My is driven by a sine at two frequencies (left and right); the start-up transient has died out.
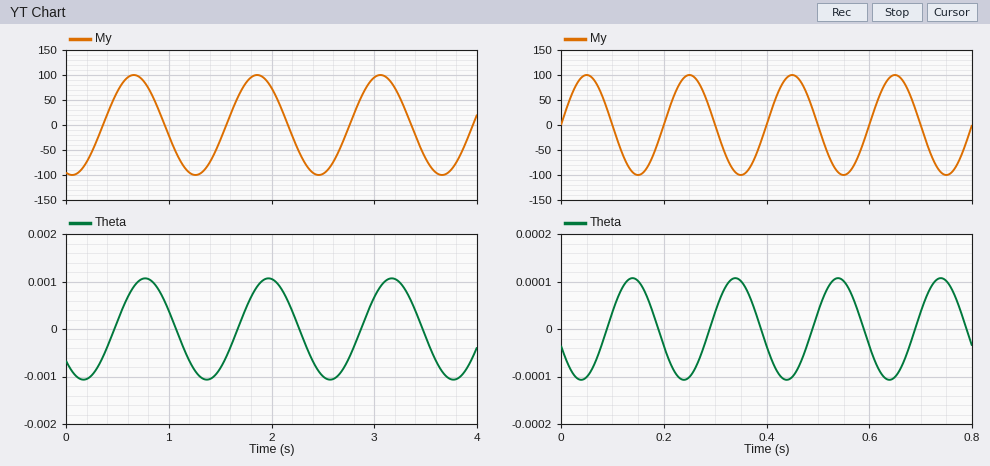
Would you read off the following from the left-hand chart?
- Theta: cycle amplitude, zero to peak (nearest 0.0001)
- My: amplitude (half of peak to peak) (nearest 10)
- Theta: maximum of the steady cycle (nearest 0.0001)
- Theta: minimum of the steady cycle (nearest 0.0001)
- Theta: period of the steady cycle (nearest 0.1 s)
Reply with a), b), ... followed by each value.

a) 0.0011
b) 100
c) 0.0011
d) -0.0011
e) 1.2 s
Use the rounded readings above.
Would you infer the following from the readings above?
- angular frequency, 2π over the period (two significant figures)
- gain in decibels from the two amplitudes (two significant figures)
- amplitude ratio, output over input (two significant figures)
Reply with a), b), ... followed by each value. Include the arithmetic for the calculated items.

a) 2π / 1.2 = 5.2 rad/s
b) 20 log10(0.0011 / 100) = -99 dB
c) 0.0011 / 100 = 0.000011
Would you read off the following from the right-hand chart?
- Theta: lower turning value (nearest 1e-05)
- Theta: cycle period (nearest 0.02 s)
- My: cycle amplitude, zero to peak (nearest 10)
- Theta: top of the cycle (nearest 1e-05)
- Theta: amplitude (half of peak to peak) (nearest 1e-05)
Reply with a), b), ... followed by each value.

a) -0.00011
b) 0.20 s
c) 100
d) 0.00011
e) 0.00011
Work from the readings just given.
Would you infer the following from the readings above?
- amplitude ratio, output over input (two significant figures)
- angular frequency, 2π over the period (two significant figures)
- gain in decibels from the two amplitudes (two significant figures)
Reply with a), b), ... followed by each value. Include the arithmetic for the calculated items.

a) 0.00011 / 100 = 0.0000011
b) 2π / 0.2 = 31 rad/s
c) 20 log10(0.00011 / 100) = -120 dB
